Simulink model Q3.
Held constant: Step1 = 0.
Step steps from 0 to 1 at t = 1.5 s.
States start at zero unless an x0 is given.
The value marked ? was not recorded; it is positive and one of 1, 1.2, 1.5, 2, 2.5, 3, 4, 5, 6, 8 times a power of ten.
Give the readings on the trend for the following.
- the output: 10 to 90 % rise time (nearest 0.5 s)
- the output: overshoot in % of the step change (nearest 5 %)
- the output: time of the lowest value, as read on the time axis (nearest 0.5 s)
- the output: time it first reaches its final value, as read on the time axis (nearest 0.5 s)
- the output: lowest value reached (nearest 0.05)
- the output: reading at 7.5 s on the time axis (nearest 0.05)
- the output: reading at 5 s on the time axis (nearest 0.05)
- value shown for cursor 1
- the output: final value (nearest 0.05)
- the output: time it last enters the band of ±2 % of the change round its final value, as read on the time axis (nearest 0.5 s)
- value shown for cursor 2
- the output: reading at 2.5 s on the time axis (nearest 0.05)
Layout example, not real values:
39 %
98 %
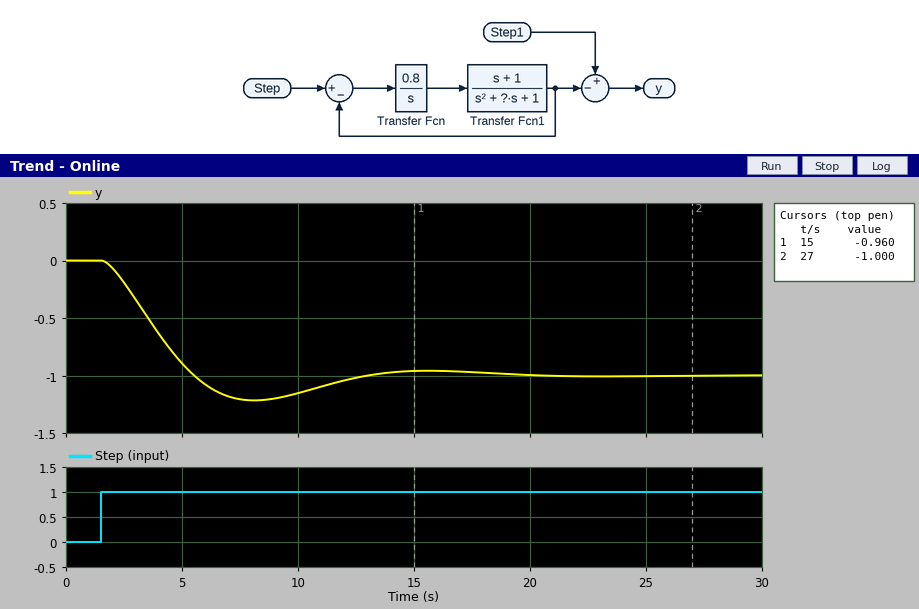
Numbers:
3.0 s
20 %
8.0 s
5.5 s
-1.20
-1.20
-0.90
-0.960
-1.00
18.5 s
-1.000
-0.20
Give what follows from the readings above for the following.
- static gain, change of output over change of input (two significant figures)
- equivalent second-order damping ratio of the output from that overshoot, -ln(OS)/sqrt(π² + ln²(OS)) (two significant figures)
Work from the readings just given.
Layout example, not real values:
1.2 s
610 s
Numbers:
-1.0
0.46
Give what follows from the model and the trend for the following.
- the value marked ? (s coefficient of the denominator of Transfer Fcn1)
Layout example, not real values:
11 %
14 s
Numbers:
4
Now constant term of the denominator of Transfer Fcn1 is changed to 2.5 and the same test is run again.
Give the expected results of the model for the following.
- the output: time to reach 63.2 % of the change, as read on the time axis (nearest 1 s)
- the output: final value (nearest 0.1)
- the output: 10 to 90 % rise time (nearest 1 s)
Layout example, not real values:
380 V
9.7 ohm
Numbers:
5 s
-1.0
6 s
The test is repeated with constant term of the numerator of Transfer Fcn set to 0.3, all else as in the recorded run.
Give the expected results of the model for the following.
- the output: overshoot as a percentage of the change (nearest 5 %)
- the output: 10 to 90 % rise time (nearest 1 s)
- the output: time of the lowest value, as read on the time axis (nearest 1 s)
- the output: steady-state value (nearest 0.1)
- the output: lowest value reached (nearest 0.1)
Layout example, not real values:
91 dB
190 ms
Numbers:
10 %
6 s
14 s
-1.0
-1.1
